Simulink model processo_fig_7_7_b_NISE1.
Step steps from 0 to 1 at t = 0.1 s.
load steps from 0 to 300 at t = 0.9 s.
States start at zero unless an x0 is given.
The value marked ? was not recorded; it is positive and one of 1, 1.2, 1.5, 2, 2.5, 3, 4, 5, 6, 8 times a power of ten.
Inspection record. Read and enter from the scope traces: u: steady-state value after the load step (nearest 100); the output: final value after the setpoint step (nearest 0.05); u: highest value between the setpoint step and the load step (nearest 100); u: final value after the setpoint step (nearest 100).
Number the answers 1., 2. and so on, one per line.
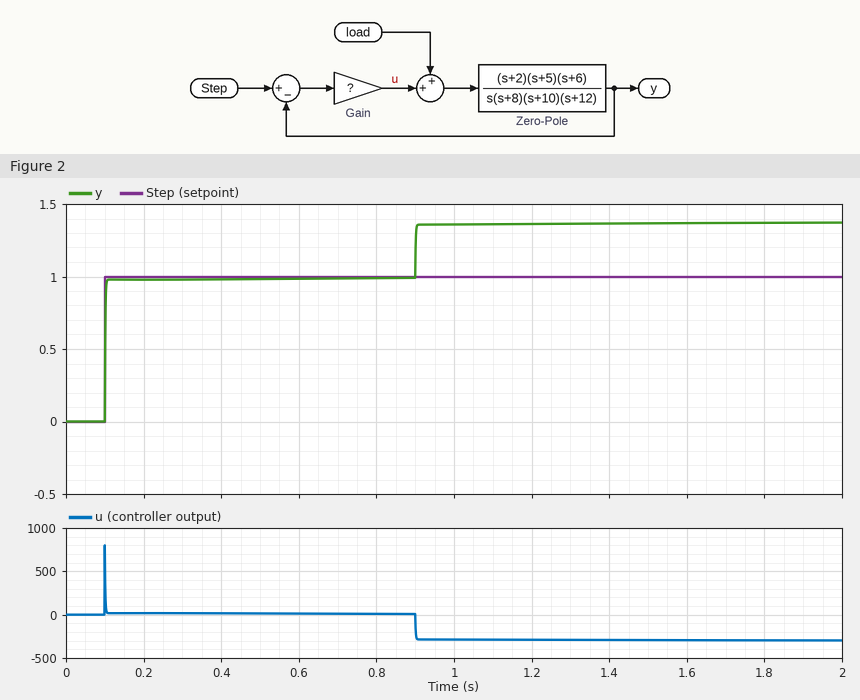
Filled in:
1. -300
2. 1.00
3. 800
4. 0
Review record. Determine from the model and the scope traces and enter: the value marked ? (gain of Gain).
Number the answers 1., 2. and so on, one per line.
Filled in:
1. 800
